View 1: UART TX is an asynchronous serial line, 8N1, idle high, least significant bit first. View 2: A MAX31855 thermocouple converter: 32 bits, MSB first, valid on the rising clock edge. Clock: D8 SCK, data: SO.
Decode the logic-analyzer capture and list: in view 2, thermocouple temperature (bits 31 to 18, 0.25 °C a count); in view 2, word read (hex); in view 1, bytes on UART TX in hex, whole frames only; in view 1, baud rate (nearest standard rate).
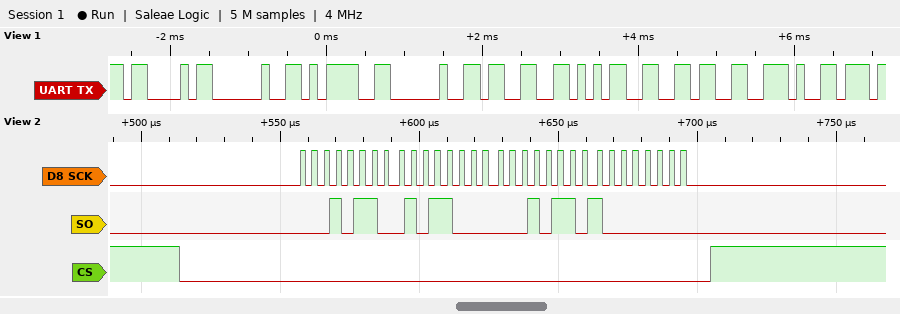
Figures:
357.50 °C
0x16581680
43 20 3D 20 33 35 36 2E
9600 baud
